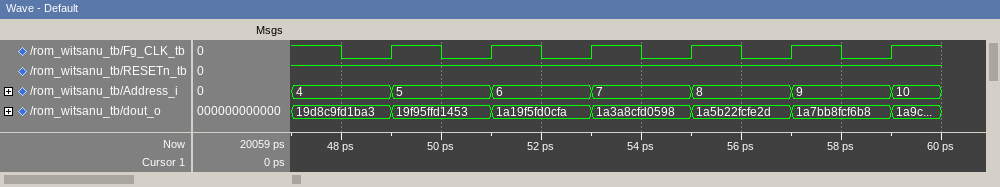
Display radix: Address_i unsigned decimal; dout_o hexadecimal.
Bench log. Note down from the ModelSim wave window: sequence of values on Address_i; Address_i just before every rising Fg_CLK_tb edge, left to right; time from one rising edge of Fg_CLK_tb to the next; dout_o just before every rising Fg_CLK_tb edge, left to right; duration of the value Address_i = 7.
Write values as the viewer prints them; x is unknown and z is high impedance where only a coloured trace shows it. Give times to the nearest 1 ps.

4, 5, 6, 7, 8, 9, 10
4, 5, 6, 7, 8, 9
2 ps
19d8c9fd1ba3, 19f95ffd1453, 1a19f5fd0cfa, 1a3a8cfd0598, 1a5b22fcfe2d, 1a7bb8fcf6b8
2 ps
